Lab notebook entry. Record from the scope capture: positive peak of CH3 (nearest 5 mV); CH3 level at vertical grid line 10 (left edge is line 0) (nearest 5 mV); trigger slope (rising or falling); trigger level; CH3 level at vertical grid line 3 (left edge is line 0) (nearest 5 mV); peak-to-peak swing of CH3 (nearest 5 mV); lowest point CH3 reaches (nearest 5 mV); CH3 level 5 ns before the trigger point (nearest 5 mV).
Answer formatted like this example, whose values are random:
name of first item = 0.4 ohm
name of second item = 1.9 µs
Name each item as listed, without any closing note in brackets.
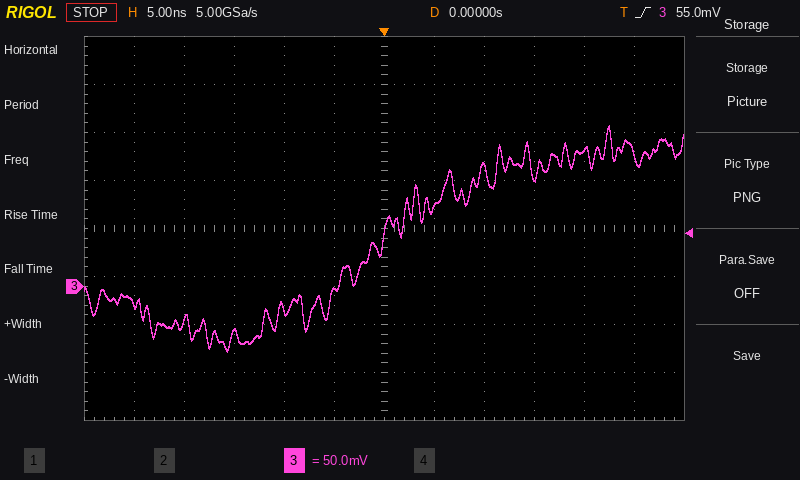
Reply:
positive peak of CH3 = 165 mV
CH3 level at vertical grid line 10 (left edge is line 0) = 140 mV
trigger slope = rising
trigger level = 55.0 mV
CH3 level at vertical grid line 3 (left edge is line 0) = -50 mV
peak-to-peak swing of CH3 = 235 mV
lowest point CH3 reaches = -70 mV
CH3 level 5 ns before the trigger point = -5 mV
